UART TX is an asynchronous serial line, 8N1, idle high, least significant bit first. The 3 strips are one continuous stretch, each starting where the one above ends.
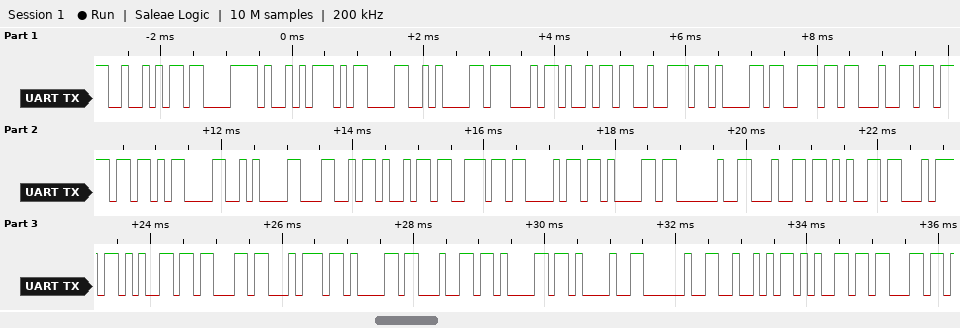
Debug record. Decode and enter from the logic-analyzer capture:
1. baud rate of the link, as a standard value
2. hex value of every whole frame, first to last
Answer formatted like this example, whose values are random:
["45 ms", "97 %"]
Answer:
["9600 baud", "52 C3 A9 0D 0A 47 69 72 61 6E 64 6F 0D 0A 4C 69 6E 68 61 20 64 65 74 65 63 74 61 64 61 21 20 52 65 63"]
